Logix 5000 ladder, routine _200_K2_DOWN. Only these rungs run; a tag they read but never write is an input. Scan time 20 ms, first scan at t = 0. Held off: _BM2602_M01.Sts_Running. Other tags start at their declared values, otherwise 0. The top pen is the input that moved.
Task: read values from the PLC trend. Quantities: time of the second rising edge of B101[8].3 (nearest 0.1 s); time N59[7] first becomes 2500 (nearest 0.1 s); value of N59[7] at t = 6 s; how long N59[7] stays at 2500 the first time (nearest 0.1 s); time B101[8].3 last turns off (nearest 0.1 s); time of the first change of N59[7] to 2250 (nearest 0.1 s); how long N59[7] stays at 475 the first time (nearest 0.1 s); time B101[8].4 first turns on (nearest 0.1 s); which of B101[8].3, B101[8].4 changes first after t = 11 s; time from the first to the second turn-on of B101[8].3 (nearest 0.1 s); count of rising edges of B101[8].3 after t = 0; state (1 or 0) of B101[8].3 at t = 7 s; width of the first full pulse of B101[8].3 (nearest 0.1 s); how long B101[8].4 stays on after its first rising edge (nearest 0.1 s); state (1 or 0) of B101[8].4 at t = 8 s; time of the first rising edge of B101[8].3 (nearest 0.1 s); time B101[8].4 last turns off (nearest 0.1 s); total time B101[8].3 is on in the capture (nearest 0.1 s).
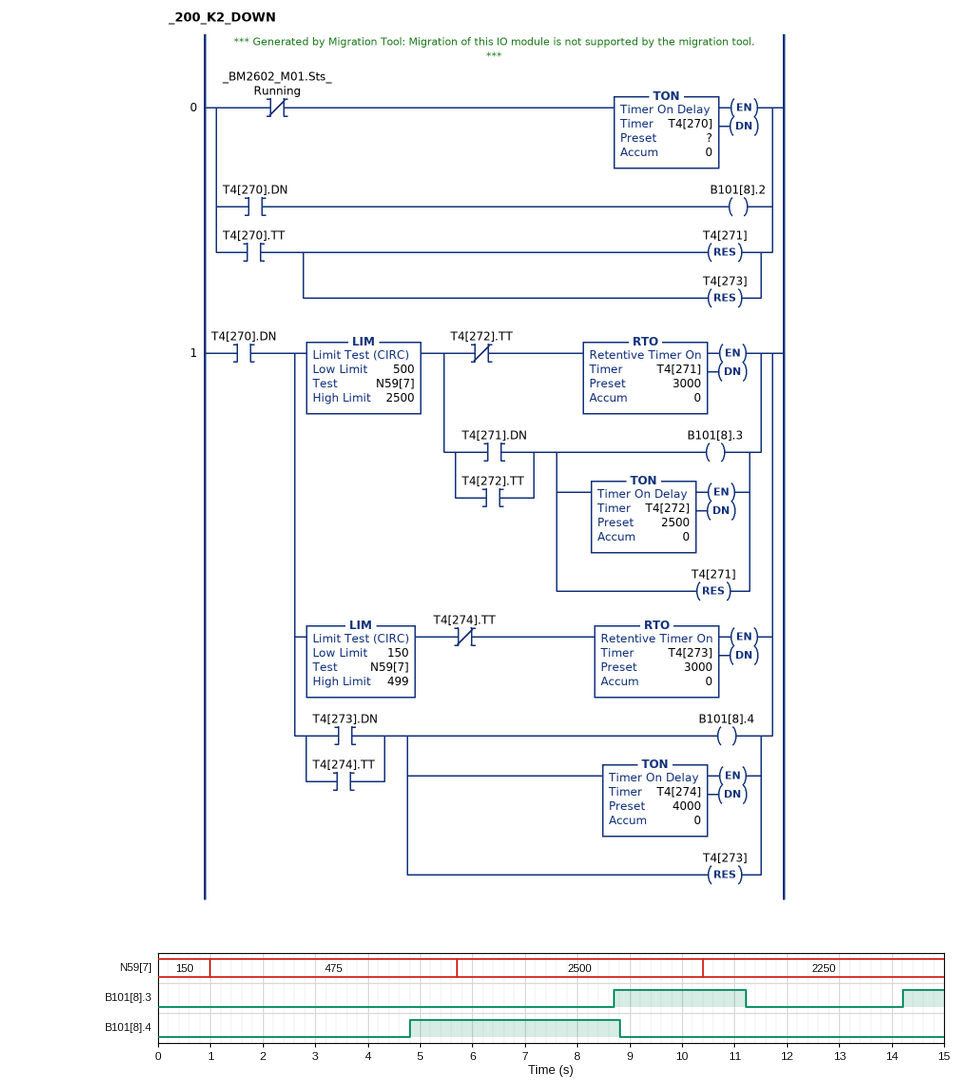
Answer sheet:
14.2 s
5.7 s
2500
4.7 s
11.2 s
10.4 s
4.7 s
4.8 s
B101[8].3
5.5 s
2
0
2.5 s
4.0 s
1
8.7 s
8.8 s
3.3 s
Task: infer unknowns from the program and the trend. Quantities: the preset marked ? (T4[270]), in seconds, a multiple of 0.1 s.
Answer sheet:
1.8 s
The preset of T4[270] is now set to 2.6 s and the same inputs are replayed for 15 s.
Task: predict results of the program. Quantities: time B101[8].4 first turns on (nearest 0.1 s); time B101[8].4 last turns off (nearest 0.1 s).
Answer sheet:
5.6 s
9.6 s
